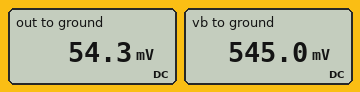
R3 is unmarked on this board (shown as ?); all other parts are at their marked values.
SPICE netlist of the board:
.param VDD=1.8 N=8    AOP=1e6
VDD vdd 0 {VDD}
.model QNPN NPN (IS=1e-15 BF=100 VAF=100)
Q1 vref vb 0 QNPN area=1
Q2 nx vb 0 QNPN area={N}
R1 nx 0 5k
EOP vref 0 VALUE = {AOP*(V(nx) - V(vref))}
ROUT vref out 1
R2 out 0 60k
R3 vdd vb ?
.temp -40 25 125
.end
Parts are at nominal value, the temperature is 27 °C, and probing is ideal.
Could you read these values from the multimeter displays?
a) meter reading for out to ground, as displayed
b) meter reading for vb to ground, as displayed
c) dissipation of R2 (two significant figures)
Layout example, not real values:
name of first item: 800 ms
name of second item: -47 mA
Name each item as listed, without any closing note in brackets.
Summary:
meter reading for out to ground, as displayed: 54.3 mV
meter reading for vb to ground, as displayed: 545.0 mV
dissipation of R2: 49 nW
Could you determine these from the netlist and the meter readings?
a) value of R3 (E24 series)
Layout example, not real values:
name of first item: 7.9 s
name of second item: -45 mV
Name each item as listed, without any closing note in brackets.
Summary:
value of R3: 110 kΩ
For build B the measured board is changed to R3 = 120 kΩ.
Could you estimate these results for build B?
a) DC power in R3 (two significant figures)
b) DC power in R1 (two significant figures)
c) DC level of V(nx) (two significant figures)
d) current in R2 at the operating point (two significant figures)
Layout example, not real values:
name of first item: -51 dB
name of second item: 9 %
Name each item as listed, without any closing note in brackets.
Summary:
DC power in R3: 13 µW
DC power in R1: 560 nW
DC level of V(nx): 53 mV
current in R2 at the operating point: 880 nA
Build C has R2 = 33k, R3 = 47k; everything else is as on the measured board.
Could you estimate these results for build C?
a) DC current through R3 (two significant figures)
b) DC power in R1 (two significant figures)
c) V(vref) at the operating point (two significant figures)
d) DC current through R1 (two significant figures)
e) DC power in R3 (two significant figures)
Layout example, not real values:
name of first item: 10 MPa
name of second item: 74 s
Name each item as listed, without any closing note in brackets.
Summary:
DC current through R3: 26 µA
DC power in R1: 820 nW
V(vref) at the operating point: 64 mV
DC current through R1: 13 µA
DC power in R3: 32 µW
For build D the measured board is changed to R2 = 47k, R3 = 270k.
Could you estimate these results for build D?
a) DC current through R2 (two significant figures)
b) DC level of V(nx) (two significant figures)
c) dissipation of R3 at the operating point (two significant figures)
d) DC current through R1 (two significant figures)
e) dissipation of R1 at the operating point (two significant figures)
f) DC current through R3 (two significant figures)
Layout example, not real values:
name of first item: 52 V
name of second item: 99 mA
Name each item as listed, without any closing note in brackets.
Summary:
DC current through R2: 750 nA
DC level of V(nx): 35 mV
dissipation of R3 at the operating point: 6.2 µW
DC current through R1: 7.1 µA
dissipation of R1 at the operating point: 250 nW
DC current through R3: 4.8 µA
